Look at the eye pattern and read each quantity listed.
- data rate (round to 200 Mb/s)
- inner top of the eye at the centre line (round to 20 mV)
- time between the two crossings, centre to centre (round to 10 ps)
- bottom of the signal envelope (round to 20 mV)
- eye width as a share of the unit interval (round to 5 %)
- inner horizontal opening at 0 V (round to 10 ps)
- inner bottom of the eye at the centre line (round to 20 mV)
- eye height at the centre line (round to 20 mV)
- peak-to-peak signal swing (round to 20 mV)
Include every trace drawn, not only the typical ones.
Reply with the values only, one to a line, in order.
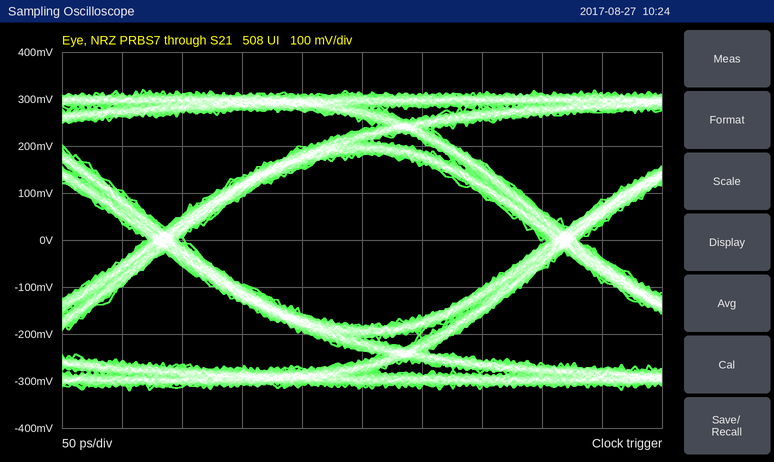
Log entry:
3.0 Gb/s
180 mV
330 ps
-320 mV
90 %
300 ps
-180 mV
360 mV
640 mV
